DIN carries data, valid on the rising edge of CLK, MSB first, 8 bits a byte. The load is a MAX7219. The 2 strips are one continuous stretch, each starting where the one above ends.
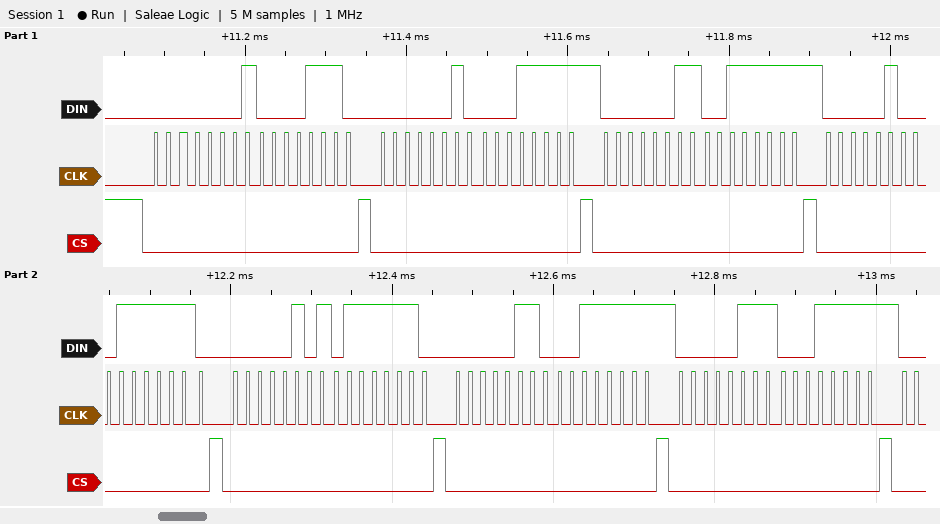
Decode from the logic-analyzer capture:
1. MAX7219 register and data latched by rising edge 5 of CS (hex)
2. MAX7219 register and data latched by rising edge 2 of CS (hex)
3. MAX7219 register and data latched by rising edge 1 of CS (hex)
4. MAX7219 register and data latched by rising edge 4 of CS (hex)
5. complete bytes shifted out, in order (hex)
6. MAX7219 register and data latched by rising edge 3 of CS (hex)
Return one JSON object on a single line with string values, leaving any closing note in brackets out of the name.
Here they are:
{"MAX7219 register and data latched by rising edge 5 of CS": "register 0x5, data 0x7E", "MAX7219 register and data latched by rising edge 2 of CS": "register 0x2, data 0x1F", "MAX7219 register and data latched by rising edge 1 of CS": "register 0x1, data 0x0E", "MAX7219 register and data latched by rising edge 4 of CS": "register 0x4, data 0x7E", "complete bytes shifted out, in order": "0x01 0x0E 0x02 0x1F 0x03 0x3F 0x04 0x7E 0x05 0x7E 0x06 0x3F 0x07 0x1F", "MAX7219 register and data latched by rising edge 3 of CS": "register 0x3, data 0x3F"}
